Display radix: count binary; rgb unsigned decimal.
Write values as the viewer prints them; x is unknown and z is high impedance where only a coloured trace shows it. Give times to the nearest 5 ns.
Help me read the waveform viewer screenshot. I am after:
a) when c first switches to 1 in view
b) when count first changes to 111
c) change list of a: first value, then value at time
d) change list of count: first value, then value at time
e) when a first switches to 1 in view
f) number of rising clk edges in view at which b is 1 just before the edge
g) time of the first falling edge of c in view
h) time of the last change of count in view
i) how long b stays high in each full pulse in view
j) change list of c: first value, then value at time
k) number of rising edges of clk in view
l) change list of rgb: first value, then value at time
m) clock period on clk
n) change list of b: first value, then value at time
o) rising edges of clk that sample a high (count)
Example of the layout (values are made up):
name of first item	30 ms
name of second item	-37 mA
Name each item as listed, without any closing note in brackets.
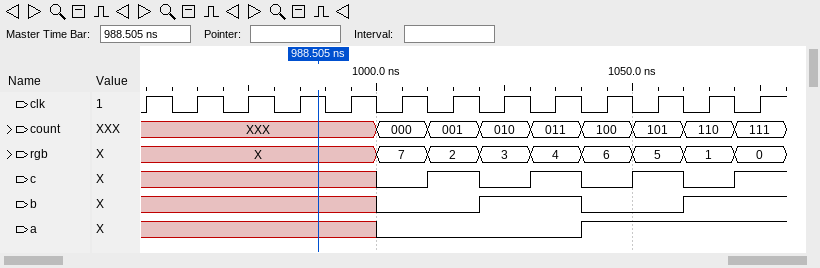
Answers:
when c first switches to 1 in view	1010 ns
when count first changes to 111	1070 ns
change list of a: first value, then value at time	x, 0 at 1000 ns, 1 at 1040 ns
change list of count: first value, then value at time	XXX, 000 at 1000 ns, 001 at 1010 ns, 010 at 1020 ns, 011 at 1030 ns, 100 at 1040 ns, 101 at 1050 ns, 110 at 1060 ns, 111 at 1070 ns
when a first switches to 1 in view	1040 ns
number of rising clk edges in view at which b is 1 just before the edge	4
time of the first falling edge of c in view	1020 ns
time of the last change of count in view	1070 ns
how long b stays high in each full pulse in view	20 ns
change list of c: first value, then value at time	x, 0 at 1000 ns, 1 at 1010 ns, 0 at 1020 ns, 1 at 1030 ns, 0 at 1040 ns, 1 at 1050 ns, 0 at 1060 ns, 1 at 1070 ns
number of rising edges of clk in view	13
change list of rgb: first value, then value at time	X, 7 at 1000 ns, 2 at 1010 ns, 3 at 1020 ns, 4 at 1030 ns, 6 at 1040 ns, 5 at 1050 ns, 1 at 1060 ns, 0 at 1070 ns
clock period on clk	10 ns
change list of b: first value, then value at time	x, 0 at 1000 ns, 1 at 1020 ns, 0 at 1040 ns, 1 at 1060 ns
rising edges of clk that sample a high	4
